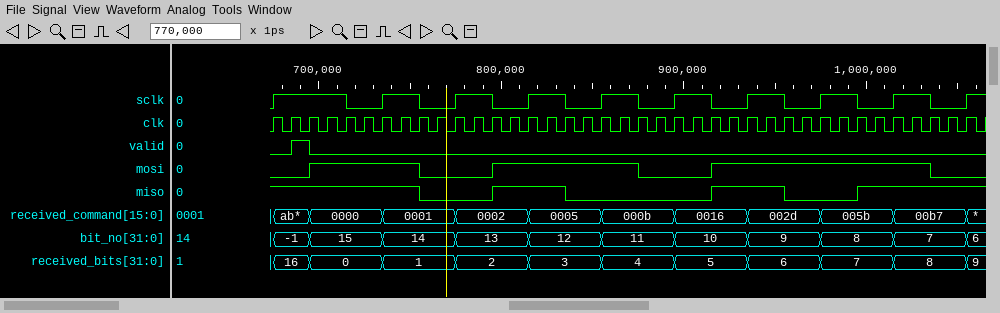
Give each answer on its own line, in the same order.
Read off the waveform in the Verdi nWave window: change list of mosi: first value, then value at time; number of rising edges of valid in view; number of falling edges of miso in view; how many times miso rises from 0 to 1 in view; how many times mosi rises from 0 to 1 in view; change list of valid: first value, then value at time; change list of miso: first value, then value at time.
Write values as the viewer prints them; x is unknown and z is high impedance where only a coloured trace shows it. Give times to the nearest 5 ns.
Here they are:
0, 1 at 695 ns, 0 at 755 ns, 1 at 795 ns, 0 at 875 ns, 1 at 915 ns, 0 at 1035 ns
1
3
3
3
0, 1 at 685 ns, 0 at 695 ns
1, 0 at 755 ns, 1 at 795 ns, 0 at 835 ns, 1 at 915 ns, 0 at 955 ns, 1 at 995 ns
